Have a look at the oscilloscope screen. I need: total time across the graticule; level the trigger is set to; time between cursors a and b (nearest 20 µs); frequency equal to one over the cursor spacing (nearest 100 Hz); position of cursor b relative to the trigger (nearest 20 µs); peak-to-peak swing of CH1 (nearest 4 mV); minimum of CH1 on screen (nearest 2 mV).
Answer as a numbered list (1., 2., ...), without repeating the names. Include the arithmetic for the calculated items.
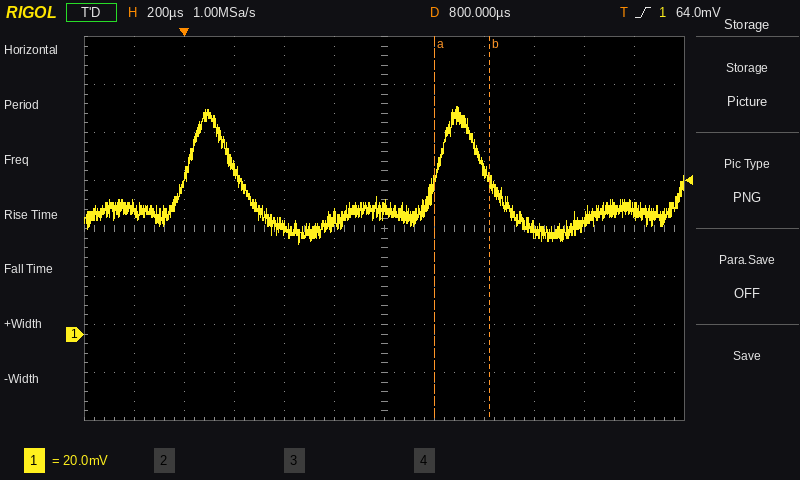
1. 2.4 ms
2. 64.0 mV
3. 220 µs
4. 1 / 220 µs ≈ 4.5 kHz
5. +1.22 ms
6. 56 mV
7. 38 mV
